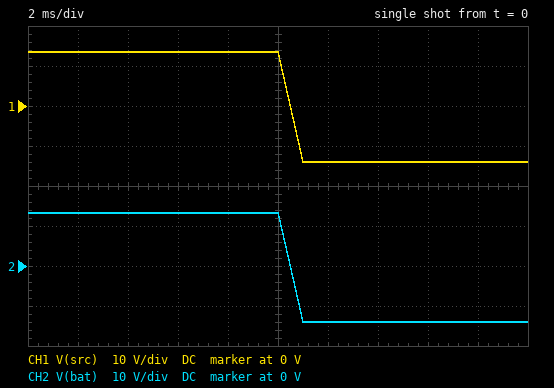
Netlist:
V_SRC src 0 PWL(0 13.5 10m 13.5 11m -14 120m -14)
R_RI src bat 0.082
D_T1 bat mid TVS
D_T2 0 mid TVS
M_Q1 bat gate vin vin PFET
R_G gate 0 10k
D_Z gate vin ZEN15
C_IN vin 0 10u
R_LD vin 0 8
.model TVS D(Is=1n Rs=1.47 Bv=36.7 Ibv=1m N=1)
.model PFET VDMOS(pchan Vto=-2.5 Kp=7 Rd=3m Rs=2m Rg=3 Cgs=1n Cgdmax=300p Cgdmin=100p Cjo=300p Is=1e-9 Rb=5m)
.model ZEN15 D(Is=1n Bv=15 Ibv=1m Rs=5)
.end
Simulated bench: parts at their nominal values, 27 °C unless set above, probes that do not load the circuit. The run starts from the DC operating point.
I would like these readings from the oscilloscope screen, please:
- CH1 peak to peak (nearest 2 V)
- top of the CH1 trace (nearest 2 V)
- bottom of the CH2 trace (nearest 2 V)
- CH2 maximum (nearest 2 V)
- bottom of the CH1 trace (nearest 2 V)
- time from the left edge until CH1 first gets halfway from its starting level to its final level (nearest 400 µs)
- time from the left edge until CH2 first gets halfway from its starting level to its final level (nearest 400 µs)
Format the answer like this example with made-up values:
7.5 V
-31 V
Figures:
28 V
14 V
-14 V
14 V
-14 V
10.4 ms
10.4 ms
